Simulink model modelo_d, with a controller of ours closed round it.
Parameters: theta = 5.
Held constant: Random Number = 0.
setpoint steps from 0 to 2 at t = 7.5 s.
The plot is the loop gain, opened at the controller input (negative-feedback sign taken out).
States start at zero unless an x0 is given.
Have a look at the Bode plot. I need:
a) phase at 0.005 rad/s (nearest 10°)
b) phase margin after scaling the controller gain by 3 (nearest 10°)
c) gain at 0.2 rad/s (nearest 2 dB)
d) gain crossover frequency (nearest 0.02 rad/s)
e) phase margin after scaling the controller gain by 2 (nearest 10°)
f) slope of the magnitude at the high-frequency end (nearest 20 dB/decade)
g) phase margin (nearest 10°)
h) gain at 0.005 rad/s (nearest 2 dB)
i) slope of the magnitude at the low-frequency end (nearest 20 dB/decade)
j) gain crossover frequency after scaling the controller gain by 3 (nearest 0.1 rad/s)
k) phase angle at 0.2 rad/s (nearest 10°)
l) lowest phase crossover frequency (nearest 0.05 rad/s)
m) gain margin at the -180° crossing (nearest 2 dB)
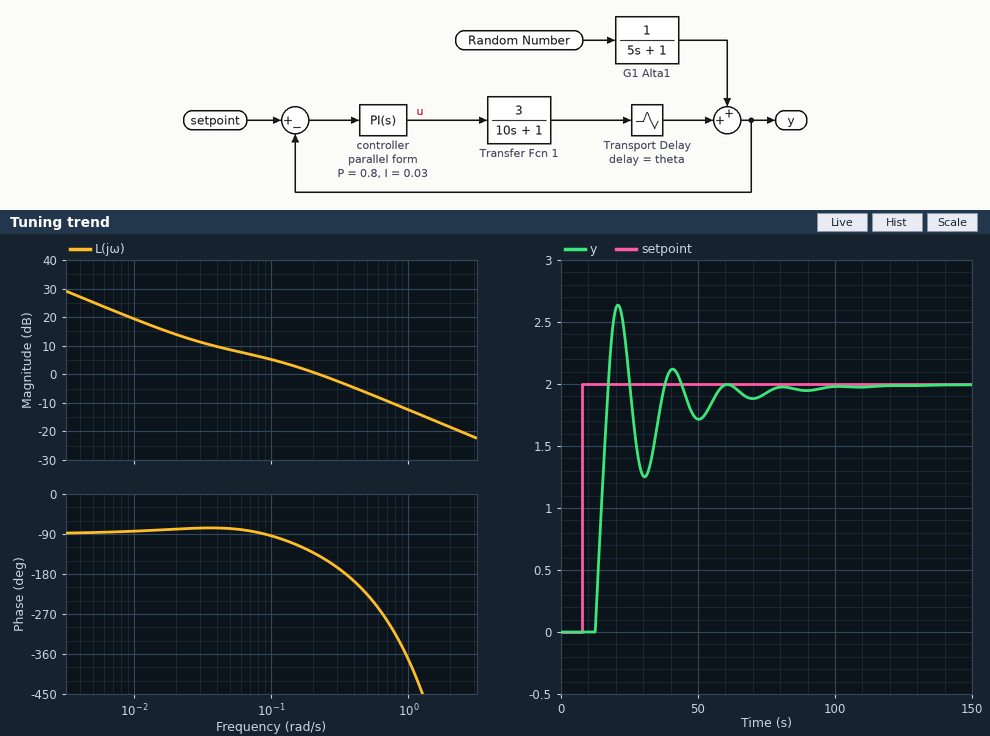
-90°
-110°
0 dB
0.22 rad/s
-40°
-20 dB/decade
40°
26 dB
-20 dB/decade
0.7 rad/s
-130°
0.35 rad/s
4 dB
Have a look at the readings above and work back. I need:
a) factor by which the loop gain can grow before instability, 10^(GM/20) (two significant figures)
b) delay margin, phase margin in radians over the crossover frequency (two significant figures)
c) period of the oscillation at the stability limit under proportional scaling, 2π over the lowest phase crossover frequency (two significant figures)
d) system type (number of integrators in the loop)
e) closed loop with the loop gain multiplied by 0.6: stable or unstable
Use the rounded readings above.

1.6
3.2 s
18 s
1
stable
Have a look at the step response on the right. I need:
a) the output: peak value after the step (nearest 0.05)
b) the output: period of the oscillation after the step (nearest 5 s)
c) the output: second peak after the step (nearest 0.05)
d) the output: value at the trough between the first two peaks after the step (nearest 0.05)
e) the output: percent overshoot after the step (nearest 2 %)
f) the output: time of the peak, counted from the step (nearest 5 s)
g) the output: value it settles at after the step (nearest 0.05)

2.65
20 s
2.10
1.25
32 %
15 s
2.00
